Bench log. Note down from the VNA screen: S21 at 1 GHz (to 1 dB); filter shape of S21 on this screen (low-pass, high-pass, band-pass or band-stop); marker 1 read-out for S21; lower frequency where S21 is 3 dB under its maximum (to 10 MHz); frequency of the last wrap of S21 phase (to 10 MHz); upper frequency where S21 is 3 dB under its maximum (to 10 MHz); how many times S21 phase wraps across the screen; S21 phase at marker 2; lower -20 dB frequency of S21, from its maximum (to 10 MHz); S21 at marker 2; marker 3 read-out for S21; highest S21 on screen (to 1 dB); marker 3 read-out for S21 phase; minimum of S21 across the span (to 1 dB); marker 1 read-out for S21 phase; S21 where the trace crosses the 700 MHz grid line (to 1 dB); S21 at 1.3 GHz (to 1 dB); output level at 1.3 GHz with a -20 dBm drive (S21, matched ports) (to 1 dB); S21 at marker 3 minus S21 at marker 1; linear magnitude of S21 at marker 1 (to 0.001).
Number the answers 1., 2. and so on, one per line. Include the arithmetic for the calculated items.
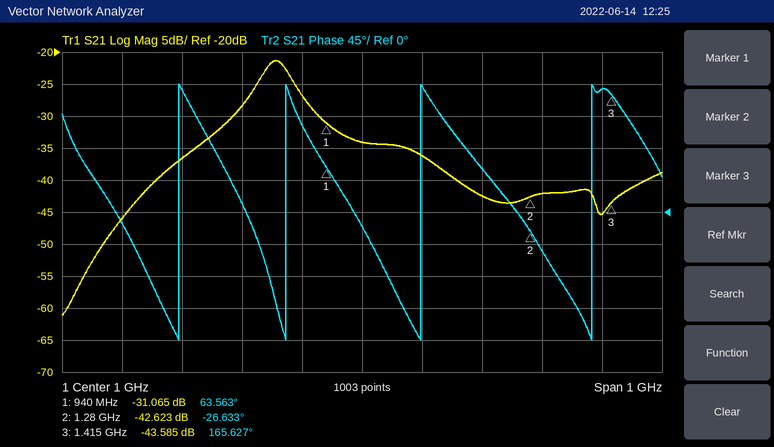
1. -34 dB
2. band-pass
3. -31.065 dB
4. 830 MHz
5. 1.38 GHz
6. 880 MHz
7. 4
8. -26.633°
9. 640 MHz
10. -42.623 dB
11. -43.585 dB
12. -21 dB
13. 165.627°
14. -61 dB
15. 63.563°
16. -37 dB
17. -42 dB
18. -20 dBm + (-42 dB) = -62 dBm
19. -43.585 − (-31.065) = -12.520 dB
20. 10^(-31.065/20) ≈ 0.028
